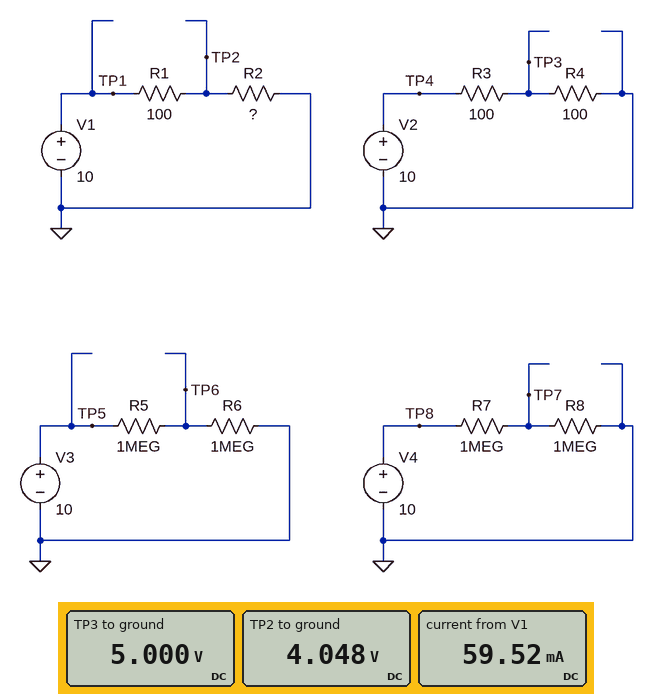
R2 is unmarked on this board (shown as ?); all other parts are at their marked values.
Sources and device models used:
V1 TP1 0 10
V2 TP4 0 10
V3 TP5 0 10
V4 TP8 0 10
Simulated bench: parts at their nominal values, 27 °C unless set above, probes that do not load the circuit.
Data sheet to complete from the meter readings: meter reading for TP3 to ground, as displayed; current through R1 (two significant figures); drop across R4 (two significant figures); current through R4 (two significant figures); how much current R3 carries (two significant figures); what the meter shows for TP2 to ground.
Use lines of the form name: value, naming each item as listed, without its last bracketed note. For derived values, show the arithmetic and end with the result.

meter reading for TP3 to ground, as displayed: 5.000 V
current through R1: (10 V - 4.048 V) / 100 Ω = 60 mA
drop across R4: 5 V = 5.0 V
current through R4: (5 V) / 100 Ω = 50 mA
how much current R3 carries: (10 V - 5 V) / 100 Ω = 50 mA
what the meter shows for TP2 to ground: 4.048 V
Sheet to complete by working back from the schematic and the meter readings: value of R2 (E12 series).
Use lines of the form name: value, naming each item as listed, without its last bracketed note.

value of R2: 68 Ω
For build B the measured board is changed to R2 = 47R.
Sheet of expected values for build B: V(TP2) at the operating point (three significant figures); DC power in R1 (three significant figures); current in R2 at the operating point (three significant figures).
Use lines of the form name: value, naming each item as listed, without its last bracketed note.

V(TP2) at the operating point: 3.20 V
DC power in R1: 463 mW
current in R2 at the operating point: 68.0 mA
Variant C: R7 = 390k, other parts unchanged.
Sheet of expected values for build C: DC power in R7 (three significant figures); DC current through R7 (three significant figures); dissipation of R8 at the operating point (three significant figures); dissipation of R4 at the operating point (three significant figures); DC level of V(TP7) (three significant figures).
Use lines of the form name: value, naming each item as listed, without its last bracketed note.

DC power in R7: 20.2 µW
DC current through R7: 7.19 µA
dissipation of R8 at the operating point: 51.8 µW
dissipation of R4 at the operating point: 250 mW
DC level of V(TP7): 7.19 V
